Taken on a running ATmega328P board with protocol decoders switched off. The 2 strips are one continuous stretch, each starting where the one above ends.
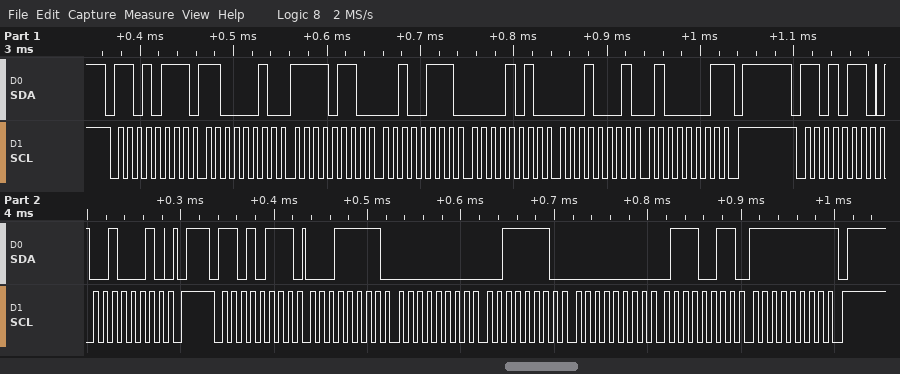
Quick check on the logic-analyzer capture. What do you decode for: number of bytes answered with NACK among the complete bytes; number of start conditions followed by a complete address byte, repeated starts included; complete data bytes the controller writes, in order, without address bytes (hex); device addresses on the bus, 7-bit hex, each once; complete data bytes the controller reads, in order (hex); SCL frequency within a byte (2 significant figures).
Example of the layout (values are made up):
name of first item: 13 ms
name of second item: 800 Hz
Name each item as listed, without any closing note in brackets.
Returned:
number of bytes answered with NACK among the complete bytes: 2
number of start conditions followed by a complete address byte, repeated starts included: 3
complete data bytes the controller writes, in order, without address bytes: 22
device addresses on the bus, 7-bit hex, each once: 0x6B
complete data bytes the controller reads, in order: C2 F6 27 0A 11 41 1F 00 3E 00 73 FF
SCL frequency within a byte: 100 kHz
